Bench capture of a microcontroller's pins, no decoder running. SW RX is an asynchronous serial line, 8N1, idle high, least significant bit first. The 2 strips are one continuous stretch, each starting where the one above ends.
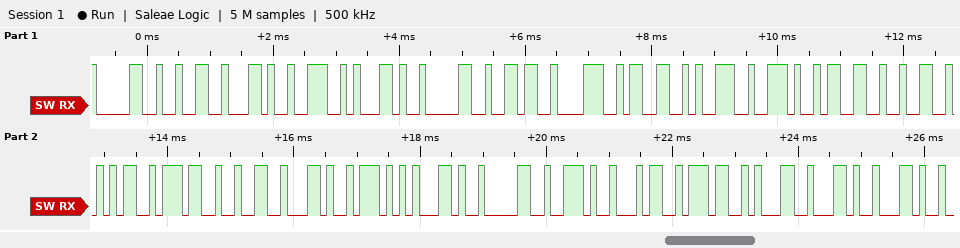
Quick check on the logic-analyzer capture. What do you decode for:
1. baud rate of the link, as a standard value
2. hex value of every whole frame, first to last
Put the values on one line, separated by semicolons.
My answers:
9600 baud; 0x30 0x32 0x2C 0x4E 0x2C 0x30 0x36 0x38 0x33 0x39 0x2E 0x33 0x32 0x35 0x37 0x32 0x2C 0x57 0x2C 0x30 0x2E 0x34 0x37 0x31 0x2C 0x2C
